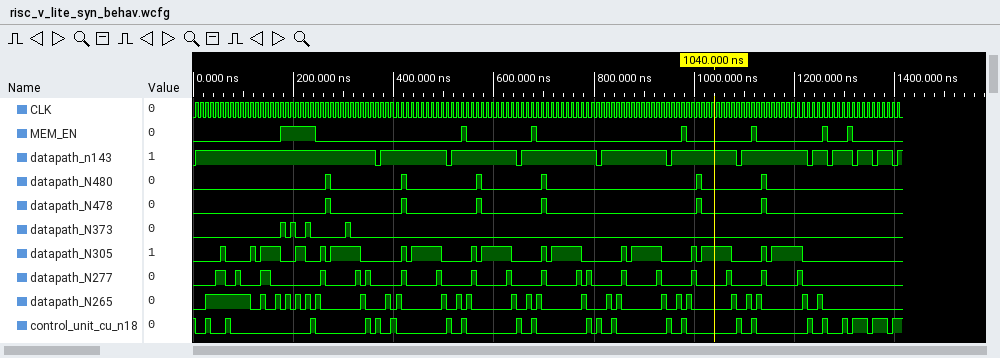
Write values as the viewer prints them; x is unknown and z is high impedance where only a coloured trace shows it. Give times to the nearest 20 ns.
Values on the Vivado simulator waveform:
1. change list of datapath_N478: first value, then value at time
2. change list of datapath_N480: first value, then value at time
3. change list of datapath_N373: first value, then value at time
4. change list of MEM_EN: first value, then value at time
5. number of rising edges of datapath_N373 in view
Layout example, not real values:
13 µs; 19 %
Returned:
0, 1 at 260 ns, 0 at 280 ns, 1 at 420 ns, 0 at 420 ns, 1 at 560 ns, 0 at 580 ns, 1 at 700 ns, 0 at 700 ns, 1 at 1000 ns, 0 at 1020 ns, 1 at 1140 ns, 0 at 1140 ns; 0, 1 at 260 ns, 0 at 280 ns, 1 at 420 ns, 0 at 420 ns, 1 at 560 ns, 0 at 580 ns, 1 at 700 ns, 0 at 700 ns, 1 at 1000 ns, 0 at 1020 ns, 1 at 1140 ns, 0 at 1140 ns; 0, 1 at 180 ns, 0 at 180 ns, 1 at 200 ns, 0 at 200 ns, 1 at 220 ns, 0 at 240 ns, 1 at 300 ns, 0 at 320 ns; 0, 1 at 180 ns, 0 at 240 ns, 1 at 540 ns, 0 at 540 ns, 1 at 680 ns, 0 at 680 ns, 1 at 980 ns, 0 at 980 ns, 1 at 1120 ns, 0 at 1120 ns, 1 at 1260 ns, 0 at 1260 ns, 1 at 1300 ns, 0 at 1320 ns; 4
